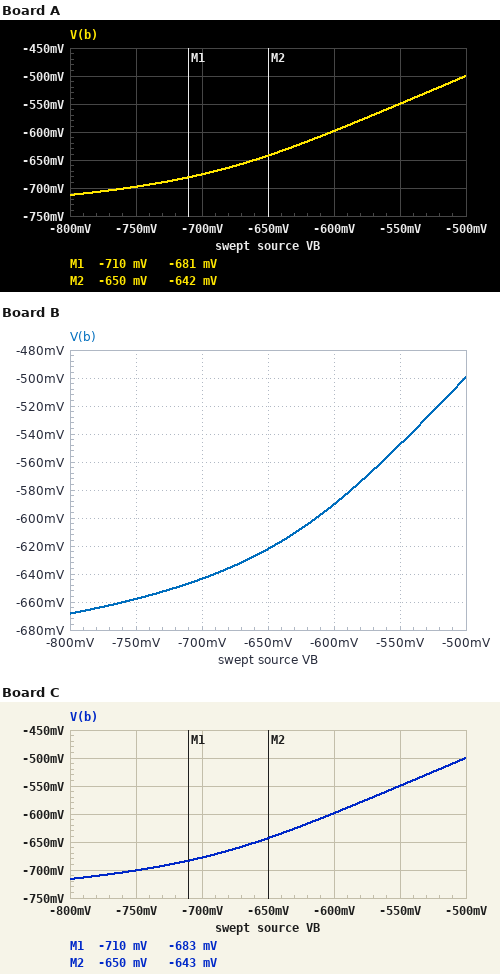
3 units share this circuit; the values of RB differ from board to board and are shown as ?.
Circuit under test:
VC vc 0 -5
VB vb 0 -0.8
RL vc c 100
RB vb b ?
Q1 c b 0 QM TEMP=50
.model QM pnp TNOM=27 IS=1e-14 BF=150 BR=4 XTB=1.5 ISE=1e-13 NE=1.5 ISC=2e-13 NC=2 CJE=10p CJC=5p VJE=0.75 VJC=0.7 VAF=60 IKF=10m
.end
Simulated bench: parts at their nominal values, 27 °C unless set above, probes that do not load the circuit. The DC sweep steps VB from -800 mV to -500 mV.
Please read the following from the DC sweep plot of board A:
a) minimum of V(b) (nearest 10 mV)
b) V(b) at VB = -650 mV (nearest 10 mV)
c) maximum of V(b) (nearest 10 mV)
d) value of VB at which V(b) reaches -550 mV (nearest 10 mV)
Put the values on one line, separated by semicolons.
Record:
-710 mV; -640 mV; -500 mV; -550 mV
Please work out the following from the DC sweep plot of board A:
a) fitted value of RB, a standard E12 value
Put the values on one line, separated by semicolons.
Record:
390 Ω
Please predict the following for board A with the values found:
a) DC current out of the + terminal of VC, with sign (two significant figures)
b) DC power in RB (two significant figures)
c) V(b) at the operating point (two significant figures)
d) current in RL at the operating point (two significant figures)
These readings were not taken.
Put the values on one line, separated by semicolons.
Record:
-15 mA; 20 µW; -710 mV; 15 mA
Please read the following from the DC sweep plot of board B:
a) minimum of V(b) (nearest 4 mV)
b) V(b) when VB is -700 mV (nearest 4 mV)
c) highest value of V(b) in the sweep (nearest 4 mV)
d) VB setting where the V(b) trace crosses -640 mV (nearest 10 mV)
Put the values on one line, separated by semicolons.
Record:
-668 mV; -644 mV; -500 mV; -690 mV
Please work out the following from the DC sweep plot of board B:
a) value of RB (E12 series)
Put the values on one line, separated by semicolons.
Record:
2.7 kΩ
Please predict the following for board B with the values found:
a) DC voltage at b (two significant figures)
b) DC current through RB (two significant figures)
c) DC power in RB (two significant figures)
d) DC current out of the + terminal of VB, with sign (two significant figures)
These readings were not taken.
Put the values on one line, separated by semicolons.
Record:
-670 mV; 49 µA; 6.4 µW; -49 µA
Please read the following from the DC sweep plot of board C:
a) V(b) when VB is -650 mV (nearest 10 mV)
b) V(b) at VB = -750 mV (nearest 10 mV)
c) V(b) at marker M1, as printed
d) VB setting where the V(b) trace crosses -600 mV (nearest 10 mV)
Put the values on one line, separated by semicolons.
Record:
-640 mV; -700 mV; -683 mV; -600 mV
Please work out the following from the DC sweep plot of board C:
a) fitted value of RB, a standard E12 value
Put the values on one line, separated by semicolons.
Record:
330 Ω
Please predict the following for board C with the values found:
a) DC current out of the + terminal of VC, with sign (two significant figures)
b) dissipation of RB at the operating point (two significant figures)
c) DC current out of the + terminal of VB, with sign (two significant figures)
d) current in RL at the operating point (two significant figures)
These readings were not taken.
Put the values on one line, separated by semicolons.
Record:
-16 mA; 21 µW; -250 µA; 16 mA
